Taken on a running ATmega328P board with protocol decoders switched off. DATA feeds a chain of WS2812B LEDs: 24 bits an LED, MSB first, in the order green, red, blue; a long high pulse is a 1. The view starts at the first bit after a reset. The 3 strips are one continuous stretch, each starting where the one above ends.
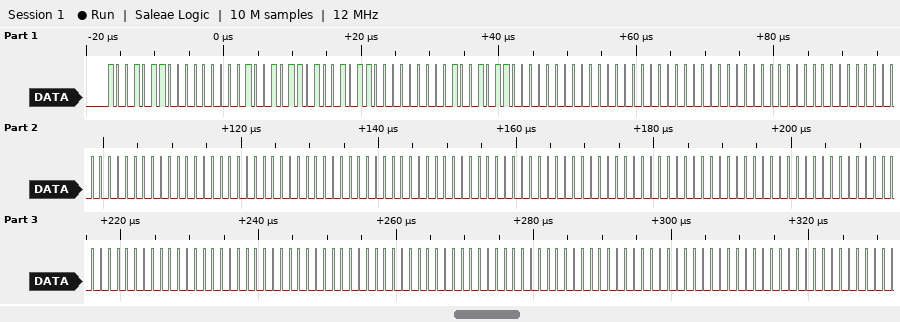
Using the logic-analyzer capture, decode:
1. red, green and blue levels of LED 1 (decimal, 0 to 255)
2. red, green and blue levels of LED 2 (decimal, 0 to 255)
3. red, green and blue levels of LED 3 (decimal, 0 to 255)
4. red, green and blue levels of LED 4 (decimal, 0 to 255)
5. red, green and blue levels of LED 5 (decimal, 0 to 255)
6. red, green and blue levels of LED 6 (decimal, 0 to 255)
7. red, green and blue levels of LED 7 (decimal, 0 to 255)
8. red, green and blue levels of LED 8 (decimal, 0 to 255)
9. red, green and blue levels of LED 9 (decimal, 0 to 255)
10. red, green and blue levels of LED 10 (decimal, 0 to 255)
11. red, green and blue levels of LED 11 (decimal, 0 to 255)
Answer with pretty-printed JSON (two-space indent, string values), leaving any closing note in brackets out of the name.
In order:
{
  "red, green and blue levels of LED 1": "0, 150, 150",
  "red, green and blue levels of LED 2": "0, 150, 150",
  "red, green and blue levels of LED 3": "0, 0, 0",
  "red, green and blue levels of LED 4": "0, 0, 0",
  "red, green and blue levels of LED 5": "0, 0, 0",
  "red, green and blue levels of LED 6": "0, 0, 0",
  "red, green and blue levels of LED 7": "0, 0, 0",
  "red, green and blue levels of LED 8": "0, 0, 0",
  "red, green and blue levels of LED 9": "0, 0, 0",
  "red, green and blue levels of LED 10": "0, 0, 0",
  "red, green and blue levels of LED 11": "0, 0, 0"
}
